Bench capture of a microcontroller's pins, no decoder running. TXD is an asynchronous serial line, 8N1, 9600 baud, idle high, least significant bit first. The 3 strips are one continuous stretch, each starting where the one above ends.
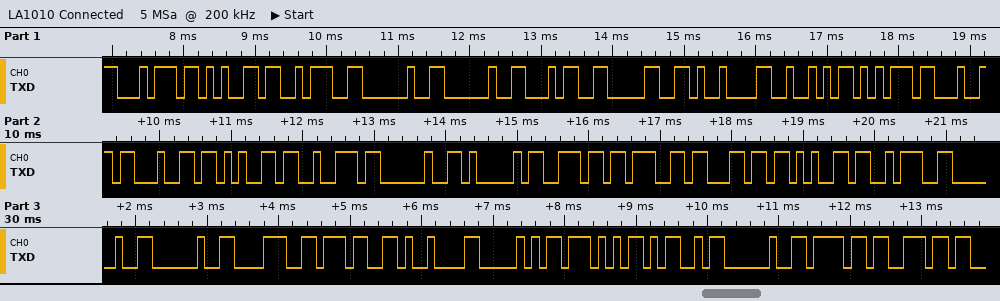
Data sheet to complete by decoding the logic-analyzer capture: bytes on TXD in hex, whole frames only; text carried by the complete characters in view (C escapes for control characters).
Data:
0x74 0x65 0x3A 0x20 0x20 0x34 0x30 0x09 0x52 0x75 0x64 0x64 0x65 0x72 0x20 0x41 0x6E 0x67 0x6C 0x65 0x3A 0x20 0x20 0x38 0x37 0x09 0x50 0x57 0x4D 0x20 0x6F 0x6E
"te:  40\tRudder Angle:  87\tPWM on"
